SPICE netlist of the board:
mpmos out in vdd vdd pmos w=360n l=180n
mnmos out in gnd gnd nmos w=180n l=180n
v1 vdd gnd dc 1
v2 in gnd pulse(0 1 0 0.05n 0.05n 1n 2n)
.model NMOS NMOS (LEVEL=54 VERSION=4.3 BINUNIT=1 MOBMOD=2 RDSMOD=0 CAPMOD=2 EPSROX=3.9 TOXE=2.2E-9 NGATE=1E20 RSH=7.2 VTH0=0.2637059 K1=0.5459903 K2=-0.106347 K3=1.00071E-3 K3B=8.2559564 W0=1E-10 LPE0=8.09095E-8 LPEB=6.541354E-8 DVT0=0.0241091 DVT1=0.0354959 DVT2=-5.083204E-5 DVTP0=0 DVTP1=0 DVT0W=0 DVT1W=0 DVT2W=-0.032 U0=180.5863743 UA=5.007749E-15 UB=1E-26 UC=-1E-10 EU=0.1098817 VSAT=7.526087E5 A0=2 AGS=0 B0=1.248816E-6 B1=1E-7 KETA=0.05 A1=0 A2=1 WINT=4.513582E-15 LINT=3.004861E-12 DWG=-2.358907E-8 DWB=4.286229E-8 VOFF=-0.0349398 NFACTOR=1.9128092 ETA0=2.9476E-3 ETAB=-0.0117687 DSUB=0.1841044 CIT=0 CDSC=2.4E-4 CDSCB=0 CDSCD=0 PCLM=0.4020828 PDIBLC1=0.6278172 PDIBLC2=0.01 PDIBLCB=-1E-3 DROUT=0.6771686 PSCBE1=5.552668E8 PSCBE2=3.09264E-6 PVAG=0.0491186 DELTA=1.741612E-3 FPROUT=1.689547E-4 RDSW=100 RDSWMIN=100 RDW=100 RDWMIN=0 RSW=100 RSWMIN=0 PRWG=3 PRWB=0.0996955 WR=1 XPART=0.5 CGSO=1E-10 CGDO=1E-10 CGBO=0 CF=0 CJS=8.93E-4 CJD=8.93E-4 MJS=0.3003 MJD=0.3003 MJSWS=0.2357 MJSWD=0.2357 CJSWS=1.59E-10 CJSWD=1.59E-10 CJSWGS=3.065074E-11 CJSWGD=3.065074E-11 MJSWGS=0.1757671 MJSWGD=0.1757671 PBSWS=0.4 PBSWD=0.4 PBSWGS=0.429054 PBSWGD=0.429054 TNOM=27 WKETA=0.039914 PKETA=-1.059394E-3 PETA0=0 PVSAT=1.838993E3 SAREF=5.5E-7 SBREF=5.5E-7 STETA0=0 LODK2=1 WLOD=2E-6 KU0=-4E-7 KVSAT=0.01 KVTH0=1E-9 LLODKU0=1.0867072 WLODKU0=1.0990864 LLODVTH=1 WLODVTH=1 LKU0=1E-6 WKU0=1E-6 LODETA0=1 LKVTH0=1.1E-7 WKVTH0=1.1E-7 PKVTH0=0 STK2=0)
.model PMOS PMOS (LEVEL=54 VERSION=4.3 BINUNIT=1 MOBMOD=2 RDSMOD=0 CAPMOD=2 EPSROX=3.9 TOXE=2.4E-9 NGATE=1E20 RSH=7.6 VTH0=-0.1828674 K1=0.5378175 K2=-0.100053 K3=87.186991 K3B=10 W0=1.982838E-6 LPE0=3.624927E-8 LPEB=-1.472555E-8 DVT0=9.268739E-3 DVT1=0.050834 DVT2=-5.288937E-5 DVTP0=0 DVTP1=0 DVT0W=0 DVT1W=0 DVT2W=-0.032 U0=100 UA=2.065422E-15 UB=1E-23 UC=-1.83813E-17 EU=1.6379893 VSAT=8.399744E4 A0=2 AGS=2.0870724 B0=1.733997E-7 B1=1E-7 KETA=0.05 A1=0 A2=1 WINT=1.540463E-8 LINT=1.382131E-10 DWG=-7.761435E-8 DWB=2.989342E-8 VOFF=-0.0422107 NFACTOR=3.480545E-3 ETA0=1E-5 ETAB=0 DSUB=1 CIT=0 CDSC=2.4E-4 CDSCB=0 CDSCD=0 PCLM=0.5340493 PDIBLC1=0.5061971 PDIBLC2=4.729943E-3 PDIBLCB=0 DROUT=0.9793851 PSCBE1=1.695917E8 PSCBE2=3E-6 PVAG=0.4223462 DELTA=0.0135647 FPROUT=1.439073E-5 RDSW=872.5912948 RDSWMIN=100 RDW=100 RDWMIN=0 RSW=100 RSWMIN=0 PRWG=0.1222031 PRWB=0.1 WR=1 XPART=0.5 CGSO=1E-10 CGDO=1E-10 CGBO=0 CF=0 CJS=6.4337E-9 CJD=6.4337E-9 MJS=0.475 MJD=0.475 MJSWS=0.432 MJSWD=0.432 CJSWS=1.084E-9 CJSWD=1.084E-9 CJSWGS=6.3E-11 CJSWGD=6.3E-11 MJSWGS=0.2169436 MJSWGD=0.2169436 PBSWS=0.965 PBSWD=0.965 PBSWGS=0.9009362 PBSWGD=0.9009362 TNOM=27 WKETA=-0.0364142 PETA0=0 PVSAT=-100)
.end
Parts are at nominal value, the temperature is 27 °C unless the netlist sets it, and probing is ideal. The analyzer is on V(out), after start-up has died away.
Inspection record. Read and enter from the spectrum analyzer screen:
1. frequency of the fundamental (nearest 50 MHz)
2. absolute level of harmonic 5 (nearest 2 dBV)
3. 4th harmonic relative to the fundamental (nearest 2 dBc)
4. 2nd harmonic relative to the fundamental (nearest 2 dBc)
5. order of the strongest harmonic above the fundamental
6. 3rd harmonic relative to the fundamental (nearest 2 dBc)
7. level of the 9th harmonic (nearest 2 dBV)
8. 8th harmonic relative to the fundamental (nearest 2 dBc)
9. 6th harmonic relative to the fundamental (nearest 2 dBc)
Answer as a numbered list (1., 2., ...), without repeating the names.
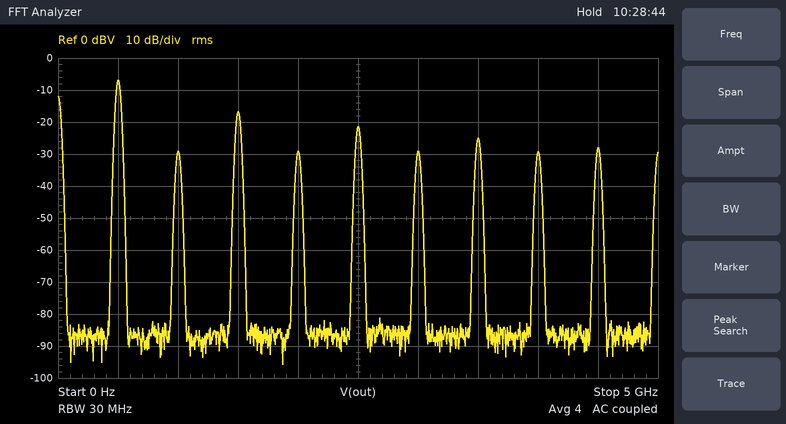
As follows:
1. 500 MHz
2. -22 dBV
3. -22 dBc
4. -22 dBc
5. 3
6. -10 dBc
7. -28 dBV
8. -22 dBc
9. -22 dBc
